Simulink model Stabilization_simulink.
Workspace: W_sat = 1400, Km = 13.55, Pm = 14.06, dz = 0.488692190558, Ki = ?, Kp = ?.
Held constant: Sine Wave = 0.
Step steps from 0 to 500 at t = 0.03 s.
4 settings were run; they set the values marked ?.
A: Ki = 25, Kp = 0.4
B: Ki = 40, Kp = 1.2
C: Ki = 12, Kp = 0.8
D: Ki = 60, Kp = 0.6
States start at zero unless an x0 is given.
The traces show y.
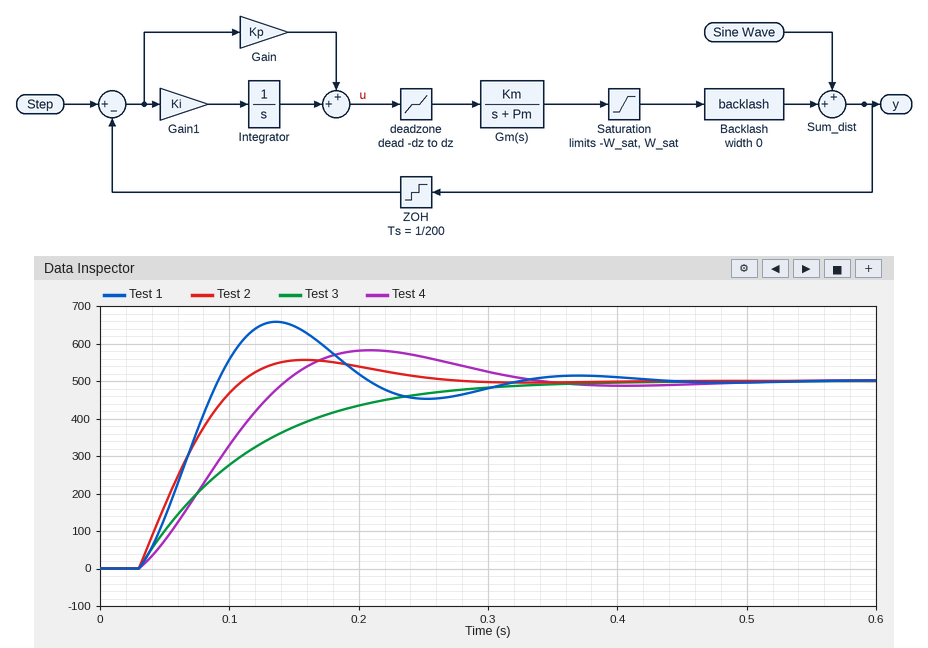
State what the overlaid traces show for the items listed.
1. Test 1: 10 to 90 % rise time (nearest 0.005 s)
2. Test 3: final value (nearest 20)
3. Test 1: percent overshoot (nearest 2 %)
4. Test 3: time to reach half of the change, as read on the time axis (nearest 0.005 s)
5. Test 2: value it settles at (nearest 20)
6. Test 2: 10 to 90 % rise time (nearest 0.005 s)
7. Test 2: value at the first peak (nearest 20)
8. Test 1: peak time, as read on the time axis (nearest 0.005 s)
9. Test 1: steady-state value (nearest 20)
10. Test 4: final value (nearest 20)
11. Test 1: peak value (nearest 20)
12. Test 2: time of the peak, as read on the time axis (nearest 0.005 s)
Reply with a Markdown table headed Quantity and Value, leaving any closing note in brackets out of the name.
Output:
| Quantity | Value |
|---|---|
| Test 1: 10 to 90 % rise time | 0.045 s |
| Test 3: final value | 500 |
| Test 1: percent overshoot | 32 % |
| Test 3: time to reach half of the change, as read on the time axis | 0.090 s |
| Test 2: value it settles at | 500 |
| Test 2: 10 to 90 % rise time | 0.060 s |
| Test 2: value at the first peak | 560 |
| Test 1: peak time, as read on the time axis | 0.135 s |
| Test 1: steady-state value | 500 |
| Test 4: final value | 500 |
| Test 1: peak value | 660 |
| Test 2: time of the peak, as read on the time axis | 0.160 s |
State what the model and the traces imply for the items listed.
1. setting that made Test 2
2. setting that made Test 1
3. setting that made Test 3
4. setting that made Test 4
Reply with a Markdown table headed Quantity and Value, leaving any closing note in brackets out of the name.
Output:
| Quantity | Value |
|---|---|
| setting that made Test 2 | B |
| setting that made Test 1 | D |
| setting that made Test 3 | C |
| setting that made Test 4 | A |
